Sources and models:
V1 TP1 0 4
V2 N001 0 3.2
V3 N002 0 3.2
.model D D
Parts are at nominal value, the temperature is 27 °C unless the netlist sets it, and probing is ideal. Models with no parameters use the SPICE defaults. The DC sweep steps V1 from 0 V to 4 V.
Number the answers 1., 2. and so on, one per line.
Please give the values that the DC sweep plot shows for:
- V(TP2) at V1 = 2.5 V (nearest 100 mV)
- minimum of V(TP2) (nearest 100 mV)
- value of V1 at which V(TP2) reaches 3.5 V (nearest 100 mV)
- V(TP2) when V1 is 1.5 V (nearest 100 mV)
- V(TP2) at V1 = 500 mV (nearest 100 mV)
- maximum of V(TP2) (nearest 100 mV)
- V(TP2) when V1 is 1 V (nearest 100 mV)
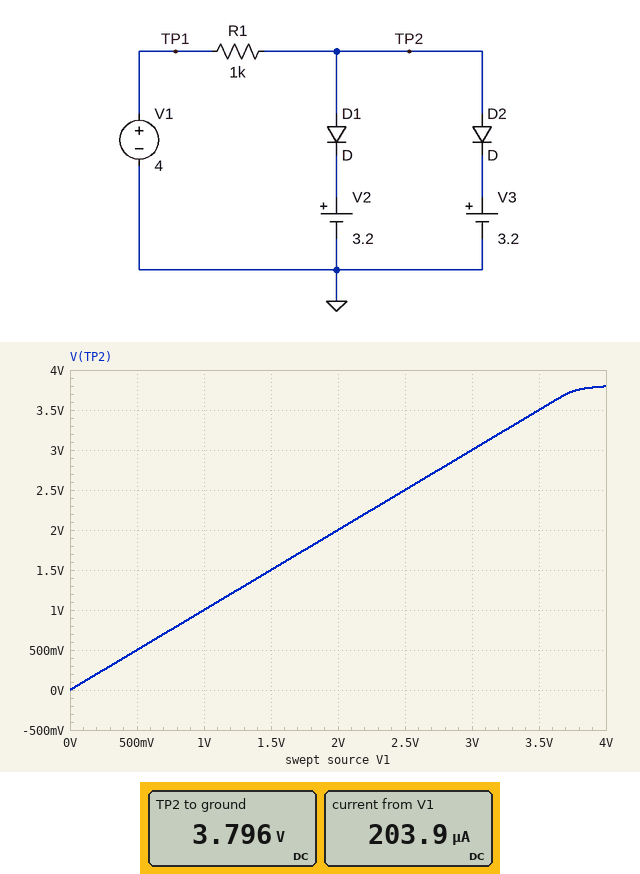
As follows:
1. 2.5 V
2. 0 V
3. 3.5 V
4. 1.5 V
5. 500 mV
6. 3.8 V
7. 1.0 V
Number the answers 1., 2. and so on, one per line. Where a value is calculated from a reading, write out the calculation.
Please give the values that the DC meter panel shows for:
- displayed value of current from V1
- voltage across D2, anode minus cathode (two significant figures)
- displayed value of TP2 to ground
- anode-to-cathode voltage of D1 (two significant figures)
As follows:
1. 203.9 µA
2. 3.796 V - 3.2 V = 600 mV
3. 3.796 V
4. 3.796 V - 3.2 V = 600 mV
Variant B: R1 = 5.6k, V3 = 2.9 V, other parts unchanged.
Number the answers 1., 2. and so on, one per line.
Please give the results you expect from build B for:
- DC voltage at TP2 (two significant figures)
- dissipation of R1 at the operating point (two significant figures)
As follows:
1. 3.5 V
2. 46 µW
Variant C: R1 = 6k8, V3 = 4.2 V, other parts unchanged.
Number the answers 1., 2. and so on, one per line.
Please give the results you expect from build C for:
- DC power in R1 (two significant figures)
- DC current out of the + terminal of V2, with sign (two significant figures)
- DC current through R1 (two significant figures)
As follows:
1. 7.9 µW
2. -34 µA
3. 34 µA
